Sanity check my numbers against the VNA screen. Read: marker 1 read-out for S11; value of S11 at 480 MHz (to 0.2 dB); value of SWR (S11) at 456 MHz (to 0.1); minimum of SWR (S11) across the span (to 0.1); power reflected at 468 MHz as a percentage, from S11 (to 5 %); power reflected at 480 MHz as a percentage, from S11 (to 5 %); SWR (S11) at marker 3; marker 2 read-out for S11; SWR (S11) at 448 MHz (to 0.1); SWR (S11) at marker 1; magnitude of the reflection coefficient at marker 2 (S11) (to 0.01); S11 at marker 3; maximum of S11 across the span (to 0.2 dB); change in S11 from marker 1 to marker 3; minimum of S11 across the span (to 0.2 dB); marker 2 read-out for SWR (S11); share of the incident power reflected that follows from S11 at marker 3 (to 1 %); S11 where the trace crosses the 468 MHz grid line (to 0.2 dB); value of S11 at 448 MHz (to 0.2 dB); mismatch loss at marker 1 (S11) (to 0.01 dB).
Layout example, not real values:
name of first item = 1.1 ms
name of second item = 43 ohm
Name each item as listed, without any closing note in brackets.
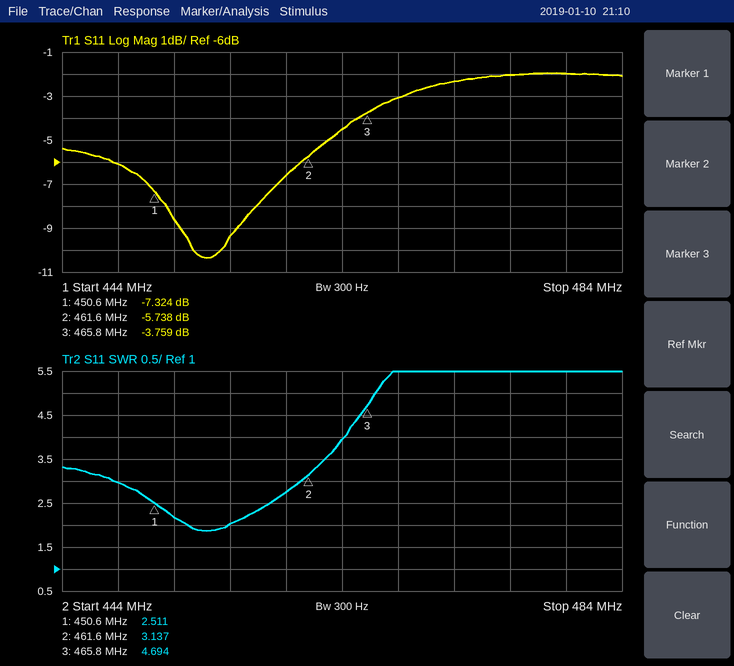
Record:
marker 1 read-out for S11 = -7.324 dB
value of S11 at 480 MHz = -2.0 dB
value of SWR (S11) at 456 MHz = 2.0
minimum of SWR (S11) across the span = 1.9
power reflected at 468 MHz as a percentage, from S11 = 50 %
power reflected at 480 MHz as a percentage, from S11 = 65 %
SWR (S11) at marker 3 = 4.694
marker 2 read-out for S11 = -5.738 dB
SWR (S11) at 448 MHz = 3.0
SWR (S11) at marker 1 = 2.511
magnitude of the reflection coefficient at marker 2 (S11) = 0.52
S11 at marker 3 = -3.759 dB
maximum of S11 across the span = -2.0 dB
change in S11 from marker 1 to marker 3 = 3.565 dB
minimum of S11 across the span = -10.4 dB
marker 2 read-out for SWR = 3.137
share of the incident power reflected that follows from S11 at marker 3 = 42 %
S11 where the trace crosses the 468 MHz grid line = -3.0 dB
value of S11 at 448 MHz = -6.0 dB
mismatch loss at marker 1 (S11) = 0.89 dB
